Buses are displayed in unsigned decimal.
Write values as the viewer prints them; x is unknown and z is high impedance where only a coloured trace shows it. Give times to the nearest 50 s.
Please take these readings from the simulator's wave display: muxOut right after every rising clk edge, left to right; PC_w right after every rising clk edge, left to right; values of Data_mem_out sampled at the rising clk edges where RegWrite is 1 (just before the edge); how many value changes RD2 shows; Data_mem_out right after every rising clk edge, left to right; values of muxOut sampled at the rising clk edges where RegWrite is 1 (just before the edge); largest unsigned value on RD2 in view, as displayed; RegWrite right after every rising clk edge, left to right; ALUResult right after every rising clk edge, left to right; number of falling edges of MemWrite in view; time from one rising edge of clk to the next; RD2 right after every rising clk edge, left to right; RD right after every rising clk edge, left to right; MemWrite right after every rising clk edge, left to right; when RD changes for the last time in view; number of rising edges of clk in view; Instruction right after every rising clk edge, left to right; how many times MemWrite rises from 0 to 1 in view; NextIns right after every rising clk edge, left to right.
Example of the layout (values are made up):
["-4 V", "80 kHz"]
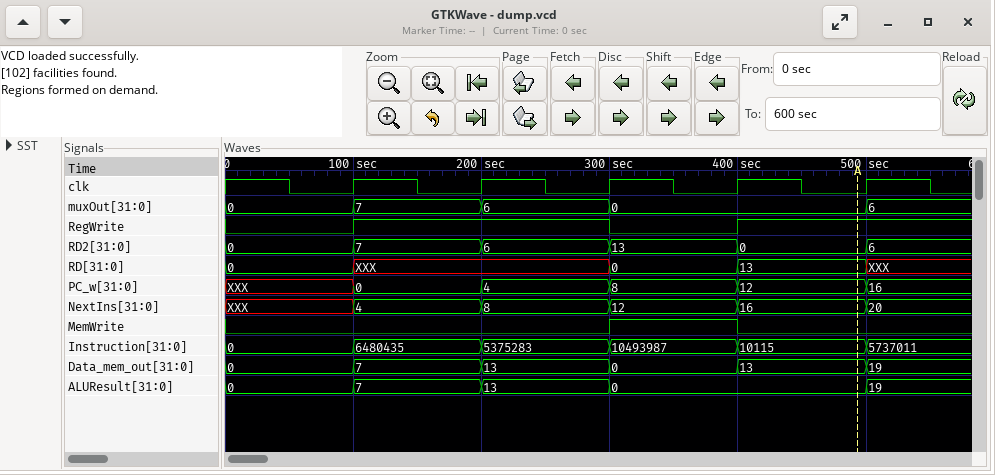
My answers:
["7, 6, 0, 0, 6", "0, 4, 8, 12, 16", "7, 13, 13", "5", "7, 13, 0, 13, 19", "7, 6, 0", "13", "1 1 0 1 1", "7, 13, 0, 0, 19", "1", "100 s", "7, 6, 13, 0, 6", "XXX, XXX, 0, 13, XXX", "0 0 1 0 0", "500 s", "5", "6480435, 5375283, 10493987, 10115, 5737011", "1", "4, 8, 12, 16, 20"]
